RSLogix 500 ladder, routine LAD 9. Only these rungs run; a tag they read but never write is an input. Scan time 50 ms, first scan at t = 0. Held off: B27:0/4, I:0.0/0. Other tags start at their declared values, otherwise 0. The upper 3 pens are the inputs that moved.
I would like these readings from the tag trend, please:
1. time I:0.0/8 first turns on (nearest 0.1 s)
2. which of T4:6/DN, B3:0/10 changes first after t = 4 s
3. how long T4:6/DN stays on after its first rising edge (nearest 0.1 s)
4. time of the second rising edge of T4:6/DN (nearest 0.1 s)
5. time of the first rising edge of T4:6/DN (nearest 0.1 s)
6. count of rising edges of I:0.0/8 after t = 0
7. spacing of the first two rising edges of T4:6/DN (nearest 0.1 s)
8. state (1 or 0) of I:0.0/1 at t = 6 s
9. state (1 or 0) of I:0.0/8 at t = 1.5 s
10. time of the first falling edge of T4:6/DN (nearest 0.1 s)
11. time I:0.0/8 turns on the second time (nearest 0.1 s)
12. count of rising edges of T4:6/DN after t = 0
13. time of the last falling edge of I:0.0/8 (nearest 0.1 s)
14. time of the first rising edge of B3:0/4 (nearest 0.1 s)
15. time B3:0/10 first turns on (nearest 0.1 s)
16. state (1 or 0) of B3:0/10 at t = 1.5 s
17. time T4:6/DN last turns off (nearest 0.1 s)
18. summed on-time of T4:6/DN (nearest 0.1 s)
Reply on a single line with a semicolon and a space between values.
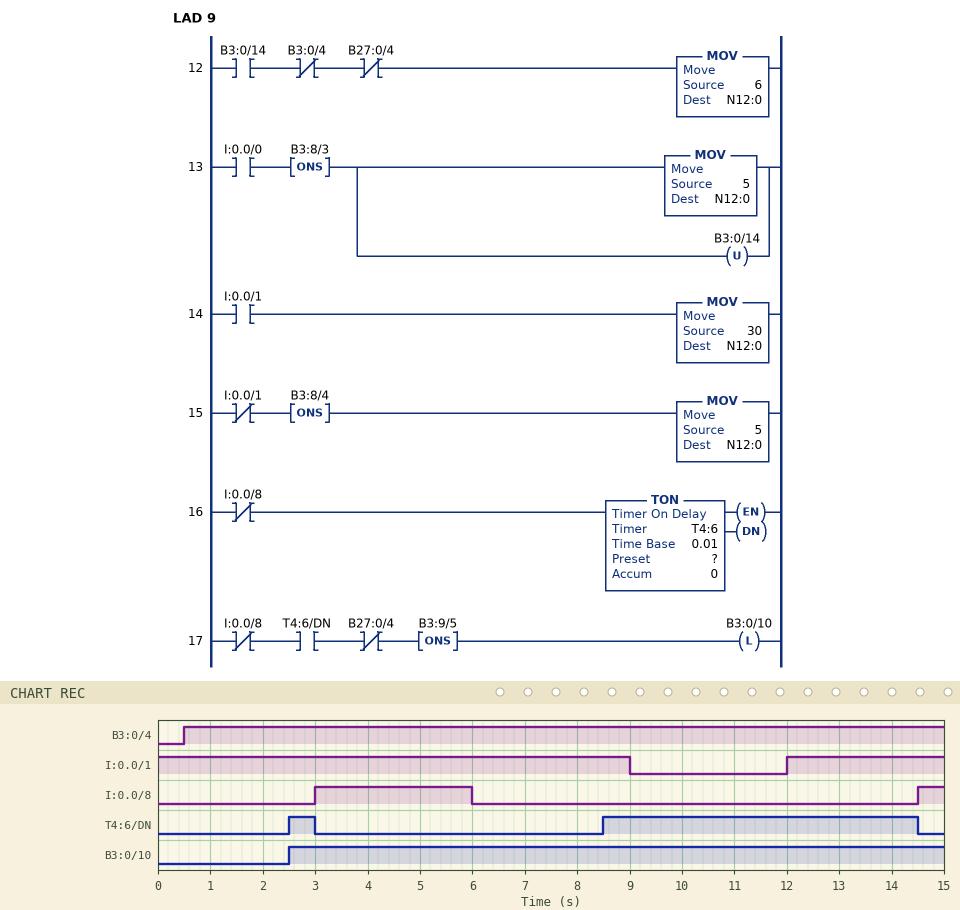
3.0 s; T4:6/DN; 0.5 s; 8.5 s; 2.5 s; 2; 6.0 s; 1; 0; 3.0 s; 14.5 s; 2; 6.0 s; 0.5 s; 2.5 s; 0; 14.5 s; 6.5 s
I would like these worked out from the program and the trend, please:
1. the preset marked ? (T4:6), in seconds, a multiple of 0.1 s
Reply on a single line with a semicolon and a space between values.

2.5 s
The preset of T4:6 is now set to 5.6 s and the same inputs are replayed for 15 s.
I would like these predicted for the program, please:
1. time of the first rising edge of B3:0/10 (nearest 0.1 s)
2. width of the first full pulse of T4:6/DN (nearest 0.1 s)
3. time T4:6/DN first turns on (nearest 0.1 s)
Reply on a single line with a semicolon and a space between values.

11.6 s; 2.9 s; 11.6 s
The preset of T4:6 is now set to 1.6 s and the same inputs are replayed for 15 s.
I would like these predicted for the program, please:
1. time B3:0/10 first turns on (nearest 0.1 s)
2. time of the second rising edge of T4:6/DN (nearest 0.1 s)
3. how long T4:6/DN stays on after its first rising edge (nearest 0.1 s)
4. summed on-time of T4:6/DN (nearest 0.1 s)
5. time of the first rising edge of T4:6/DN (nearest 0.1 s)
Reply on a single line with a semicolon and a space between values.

1.6 s; 7.6 s; 1.4 s; 8.3 s; 1.6 s
